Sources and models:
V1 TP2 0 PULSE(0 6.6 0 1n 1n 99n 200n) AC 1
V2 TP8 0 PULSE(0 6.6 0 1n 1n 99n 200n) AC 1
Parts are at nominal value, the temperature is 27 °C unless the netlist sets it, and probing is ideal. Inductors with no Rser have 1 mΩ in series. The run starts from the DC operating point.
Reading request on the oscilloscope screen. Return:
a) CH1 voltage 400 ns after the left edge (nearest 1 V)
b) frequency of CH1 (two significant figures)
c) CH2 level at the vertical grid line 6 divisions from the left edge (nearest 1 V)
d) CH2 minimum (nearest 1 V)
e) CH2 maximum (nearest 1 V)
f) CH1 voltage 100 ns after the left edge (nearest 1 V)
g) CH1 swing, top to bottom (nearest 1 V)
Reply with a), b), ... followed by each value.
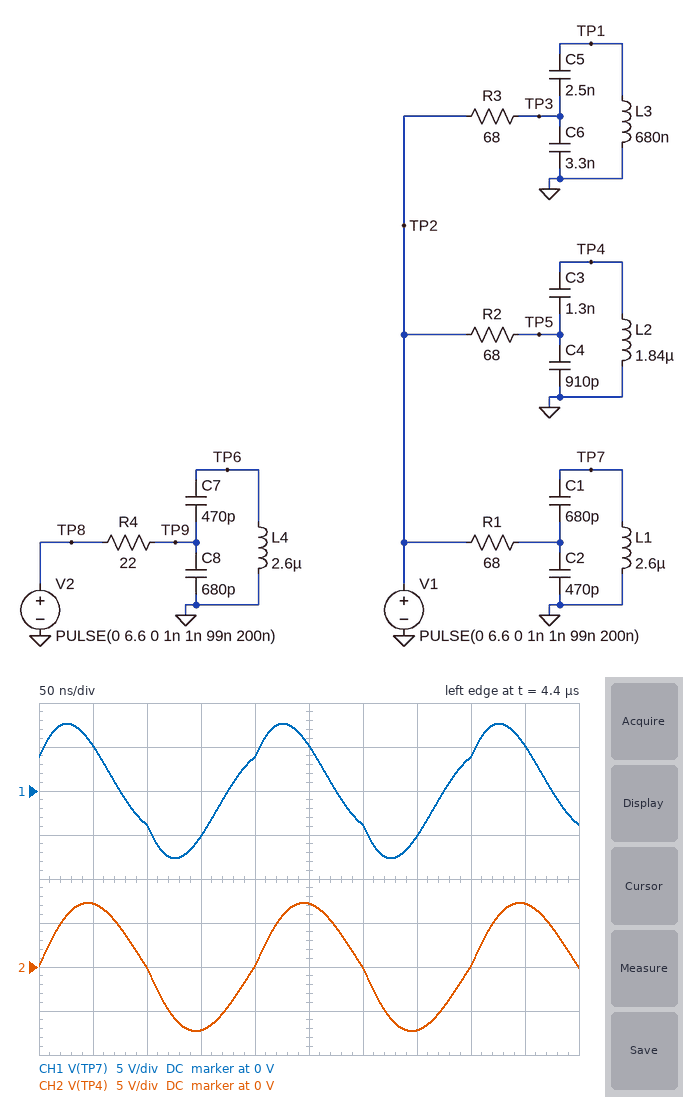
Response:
a) 4 V
b) 5.0 MHz
c) 0 V
d) -7 V
e) 7 V
f) -4 V
g) 15 V
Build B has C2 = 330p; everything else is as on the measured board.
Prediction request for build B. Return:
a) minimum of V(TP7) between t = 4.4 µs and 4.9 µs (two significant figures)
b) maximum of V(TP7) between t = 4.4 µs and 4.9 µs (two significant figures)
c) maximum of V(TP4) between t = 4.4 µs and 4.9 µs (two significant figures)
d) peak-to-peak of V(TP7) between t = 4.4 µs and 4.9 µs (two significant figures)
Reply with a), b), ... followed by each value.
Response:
a) -6.9 V
b) 6.9 V
c) 7.3 V
d) 14 V
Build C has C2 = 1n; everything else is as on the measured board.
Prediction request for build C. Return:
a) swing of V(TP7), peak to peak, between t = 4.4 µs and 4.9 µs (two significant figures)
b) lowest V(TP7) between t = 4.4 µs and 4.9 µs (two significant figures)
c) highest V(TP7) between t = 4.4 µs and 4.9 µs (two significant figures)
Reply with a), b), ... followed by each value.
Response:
a) 19 V
b) -9.6 V
c) 9.6 V
